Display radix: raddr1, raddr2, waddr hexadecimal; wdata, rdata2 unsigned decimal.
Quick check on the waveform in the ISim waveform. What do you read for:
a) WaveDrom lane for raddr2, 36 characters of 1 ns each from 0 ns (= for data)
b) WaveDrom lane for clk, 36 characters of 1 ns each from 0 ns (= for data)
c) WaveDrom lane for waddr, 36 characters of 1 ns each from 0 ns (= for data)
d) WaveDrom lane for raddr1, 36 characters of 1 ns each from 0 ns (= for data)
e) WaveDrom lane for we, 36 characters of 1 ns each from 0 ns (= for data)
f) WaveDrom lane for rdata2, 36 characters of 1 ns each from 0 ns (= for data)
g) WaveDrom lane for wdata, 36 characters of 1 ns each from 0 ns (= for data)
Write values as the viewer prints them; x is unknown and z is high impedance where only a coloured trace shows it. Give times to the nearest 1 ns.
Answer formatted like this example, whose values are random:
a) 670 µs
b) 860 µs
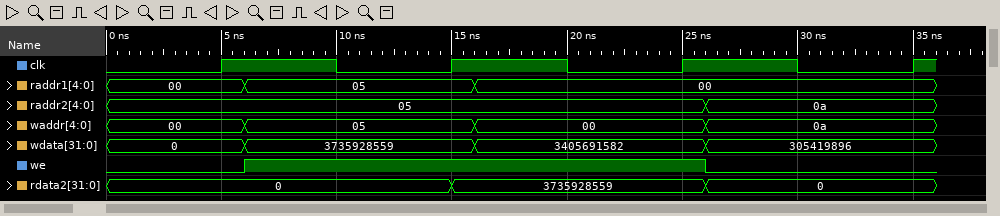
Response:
a) {name: 'raddr2', wave: '=.........................=.........', data: '05 0a'}
b) {name: 'clk', wave: '0....1....0....1....0....1....0....1'}
c) {name: 'waddr', wave: '=.....=.........=.........=.........', data: '00 05 00 0a'}
d) {name: 'raddr1', wave: '=.....=.........=...................', data: '00 05 00'}
e) {name: 'we', wave: '0.....1...................0.........'}
f) {name: 'rdata2', wave: '=..............=..........=.........', data: '0 3735928559 0'}
g) {name: 'wdata', wave: '=.....=.........=.........=.........', data: '0 3735928559 3405691582 305419896'}
